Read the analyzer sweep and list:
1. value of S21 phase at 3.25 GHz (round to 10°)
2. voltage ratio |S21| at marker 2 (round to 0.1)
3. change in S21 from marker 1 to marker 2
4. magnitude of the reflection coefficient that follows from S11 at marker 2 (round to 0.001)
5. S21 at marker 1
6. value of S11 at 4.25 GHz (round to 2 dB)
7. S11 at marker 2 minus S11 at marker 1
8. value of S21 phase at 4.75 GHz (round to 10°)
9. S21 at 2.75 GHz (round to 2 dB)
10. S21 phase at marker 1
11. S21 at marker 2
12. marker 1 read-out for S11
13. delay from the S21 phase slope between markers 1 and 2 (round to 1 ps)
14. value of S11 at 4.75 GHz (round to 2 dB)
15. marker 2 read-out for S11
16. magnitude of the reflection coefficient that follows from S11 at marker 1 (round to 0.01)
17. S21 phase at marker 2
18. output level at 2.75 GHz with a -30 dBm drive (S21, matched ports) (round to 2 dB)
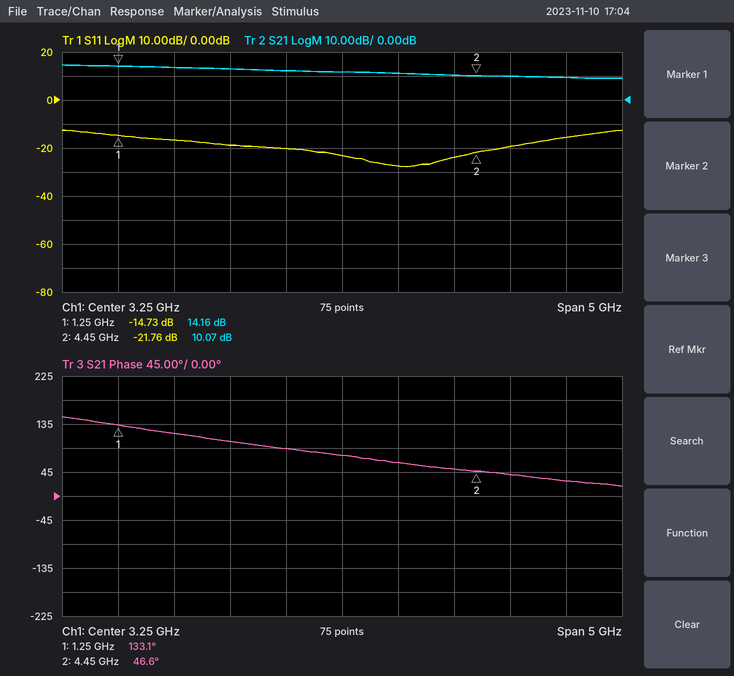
80°
3.2
-4.09 dB
0.082
14.16 dB
-24 dB
-7.03 dB
40°
12 dB
133.1°
10.07 dB
-14.73 dB
75 ps
-20 dB
-21.76 dB
0.18
46.6°
-18 dBm
